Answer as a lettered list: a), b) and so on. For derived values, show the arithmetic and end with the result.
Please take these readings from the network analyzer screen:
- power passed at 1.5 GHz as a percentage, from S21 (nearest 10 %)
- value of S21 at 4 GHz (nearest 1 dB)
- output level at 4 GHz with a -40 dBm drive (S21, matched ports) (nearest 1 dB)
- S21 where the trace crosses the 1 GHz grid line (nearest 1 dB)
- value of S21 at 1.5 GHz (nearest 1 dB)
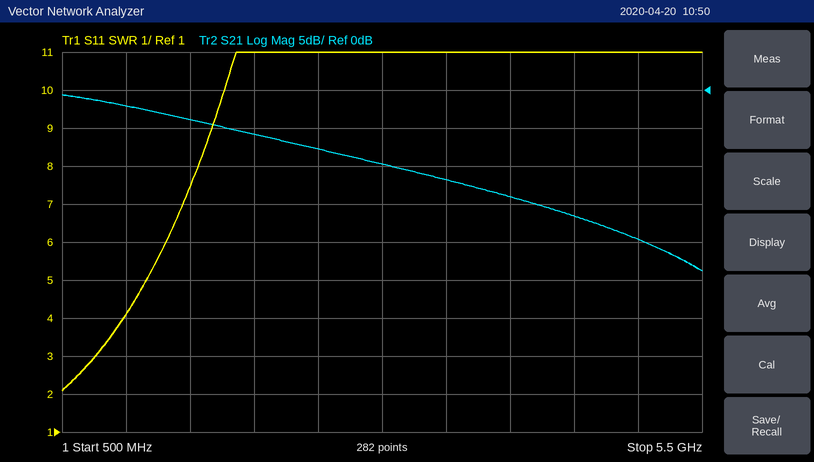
a) 10^(-4/10) ≈ 40 %
b) -14 dB
c) -40 dBm + (-14 dB) = -54 dBm
d) -2 dB
e) -4 dB
